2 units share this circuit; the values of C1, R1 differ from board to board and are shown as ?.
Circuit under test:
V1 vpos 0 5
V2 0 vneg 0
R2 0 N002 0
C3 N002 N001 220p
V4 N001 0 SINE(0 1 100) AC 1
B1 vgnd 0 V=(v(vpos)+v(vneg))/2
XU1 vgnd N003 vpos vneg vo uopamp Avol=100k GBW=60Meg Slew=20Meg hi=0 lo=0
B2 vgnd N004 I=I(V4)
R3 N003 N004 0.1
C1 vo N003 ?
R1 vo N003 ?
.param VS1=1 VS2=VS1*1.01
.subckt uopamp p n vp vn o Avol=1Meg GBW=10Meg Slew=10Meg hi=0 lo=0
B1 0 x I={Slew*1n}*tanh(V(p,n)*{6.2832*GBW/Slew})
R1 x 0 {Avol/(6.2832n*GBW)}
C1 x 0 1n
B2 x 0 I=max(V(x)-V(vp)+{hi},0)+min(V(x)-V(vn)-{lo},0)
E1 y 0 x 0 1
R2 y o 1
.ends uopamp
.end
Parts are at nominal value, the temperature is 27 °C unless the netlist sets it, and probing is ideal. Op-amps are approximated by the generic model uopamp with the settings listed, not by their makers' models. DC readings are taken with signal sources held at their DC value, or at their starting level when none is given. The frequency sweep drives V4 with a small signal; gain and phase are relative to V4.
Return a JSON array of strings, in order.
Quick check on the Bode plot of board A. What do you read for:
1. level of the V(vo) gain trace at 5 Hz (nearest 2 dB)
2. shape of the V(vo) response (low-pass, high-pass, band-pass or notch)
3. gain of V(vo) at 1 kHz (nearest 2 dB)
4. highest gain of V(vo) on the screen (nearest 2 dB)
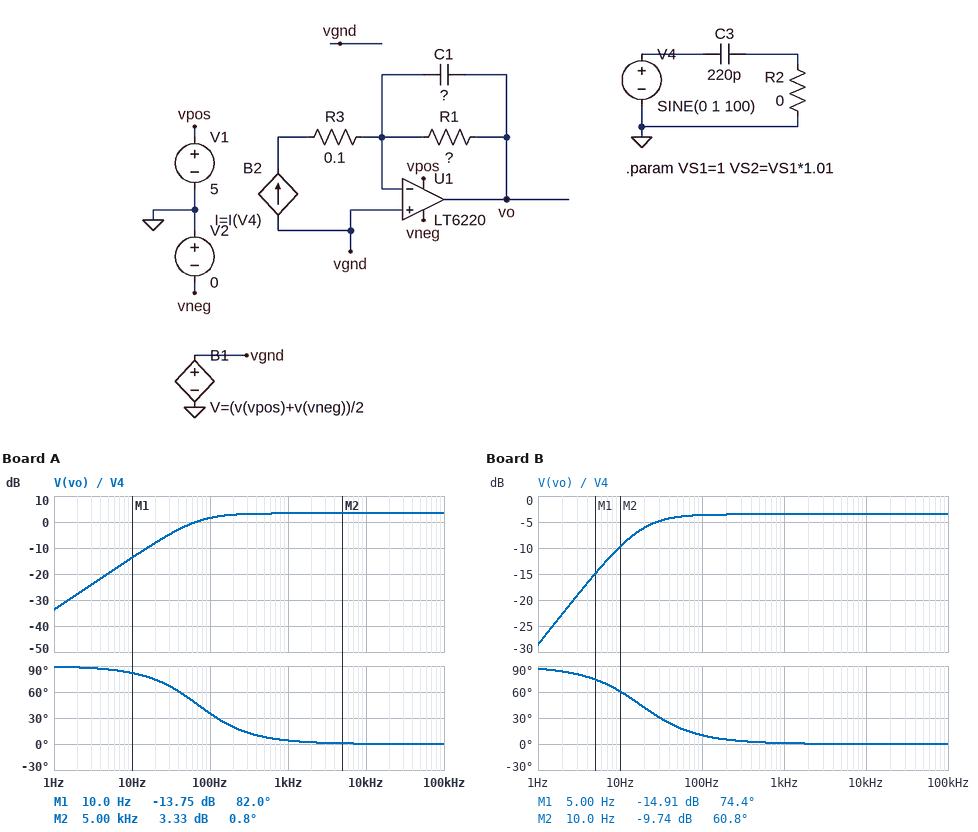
["-20 dB", "high-pass", "4 dB", "4 dB"]
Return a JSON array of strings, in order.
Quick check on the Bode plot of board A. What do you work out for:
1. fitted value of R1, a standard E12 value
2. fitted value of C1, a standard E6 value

["15 MΩ", "150 pF"]
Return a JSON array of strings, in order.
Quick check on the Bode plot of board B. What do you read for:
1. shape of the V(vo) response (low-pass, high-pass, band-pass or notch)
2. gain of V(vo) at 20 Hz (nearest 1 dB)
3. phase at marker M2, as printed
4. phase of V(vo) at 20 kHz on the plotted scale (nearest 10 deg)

["high-pass", "-6 dB", "60.8 deg", "0 deg"]
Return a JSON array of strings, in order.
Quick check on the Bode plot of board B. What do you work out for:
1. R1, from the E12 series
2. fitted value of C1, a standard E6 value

["27 MΩ", "330 pF"]
